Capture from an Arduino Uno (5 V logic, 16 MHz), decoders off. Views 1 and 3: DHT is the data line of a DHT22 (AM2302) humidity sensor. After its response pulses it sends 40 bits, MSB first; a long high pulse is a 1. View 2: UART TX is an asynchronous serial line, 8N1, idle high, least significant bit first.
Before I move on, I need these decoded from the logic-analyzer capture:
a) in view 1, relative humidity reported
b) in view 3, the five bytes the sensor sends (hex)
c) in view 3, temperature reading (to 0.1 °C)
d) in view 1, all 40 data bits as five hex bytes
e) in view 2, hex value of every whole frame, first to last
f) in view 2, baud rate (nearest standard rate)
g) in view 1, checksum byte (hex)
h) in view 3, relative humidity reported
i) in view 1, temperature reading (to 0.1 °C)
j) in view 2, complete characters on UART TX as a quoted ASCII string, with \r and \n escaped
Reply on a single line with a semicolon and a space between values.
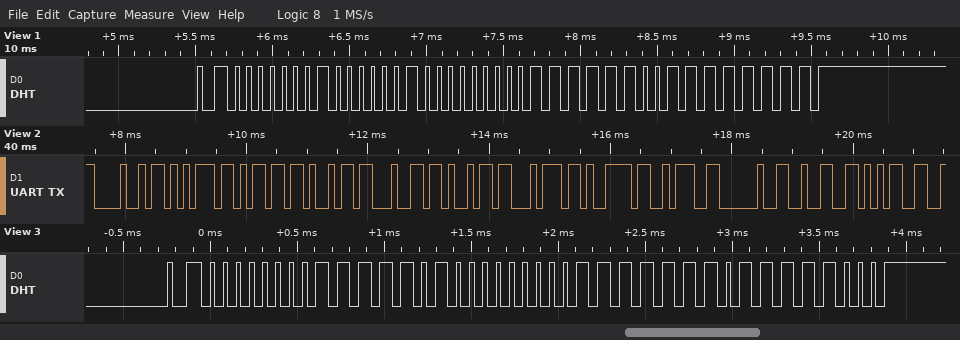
25.8 %; 00 FA 00 FE F8; 25.4 °C; 01 02 00 FC FF; 48 75 6D 69 64 69 74 79 3A 20 32 35; 9600 baud; 0xFF; 25.0 %; 25.2 °C; "Humidity: 25"
